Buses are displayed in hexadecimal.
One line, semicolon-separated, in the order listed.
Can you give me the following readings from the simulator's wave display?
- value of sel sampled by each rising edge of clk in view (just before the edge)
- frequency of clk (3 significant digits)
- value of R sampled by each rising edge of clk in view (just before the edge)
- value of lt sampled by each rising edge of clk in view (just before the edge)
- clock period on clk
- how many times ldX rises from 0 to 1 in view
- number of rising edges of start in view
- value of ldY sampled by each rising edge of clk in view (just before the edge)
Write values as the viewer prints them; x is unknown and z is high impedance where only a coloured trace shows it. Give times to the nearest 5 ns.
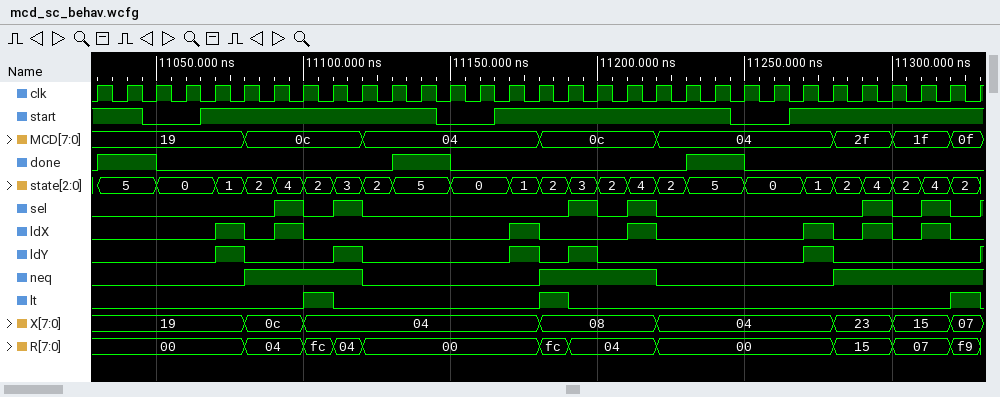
0 0 0 0 0 0 0 1 0 1 0 0 0 0 0 0 0 1 0 1 0 0 0 0 0 0 0 1 0 1 0; 100 MHz; 00, 00, 00, 00, 00, 00, 04, 04, fc, 04, 00, 00, 00, 00, 00, 00, fc, 04, 04, 04, 00, 00, 00, 00, 00, 00, 15, 15, 07, 07, f9; 0 0 0 0 0 0 0 0 1 0 0 0 0 0 0 0 1 0 0 0 0 0 0 0 0 0 0 0 0 0 1; 10 ns; 7; 3; 0 0 0 0 0 1 0 0 0 1 0 0 0 0 0 1 0 1 0 0 0 0 0 0 0 1 0 0 0 0 0
